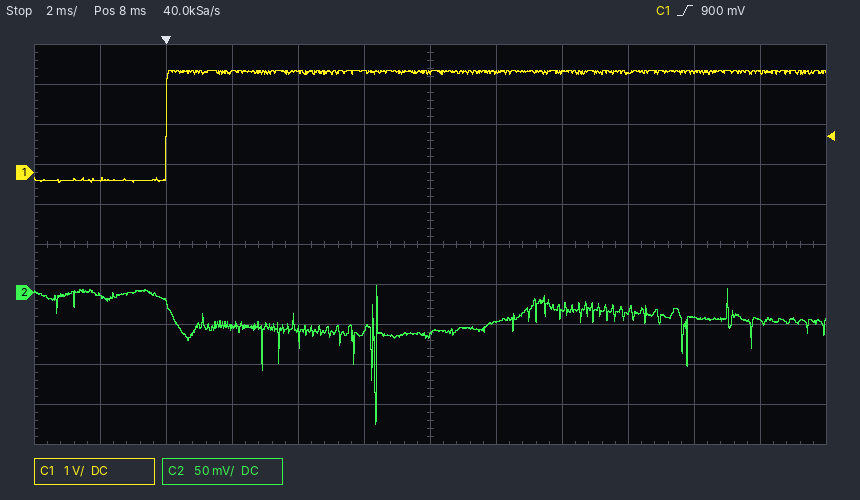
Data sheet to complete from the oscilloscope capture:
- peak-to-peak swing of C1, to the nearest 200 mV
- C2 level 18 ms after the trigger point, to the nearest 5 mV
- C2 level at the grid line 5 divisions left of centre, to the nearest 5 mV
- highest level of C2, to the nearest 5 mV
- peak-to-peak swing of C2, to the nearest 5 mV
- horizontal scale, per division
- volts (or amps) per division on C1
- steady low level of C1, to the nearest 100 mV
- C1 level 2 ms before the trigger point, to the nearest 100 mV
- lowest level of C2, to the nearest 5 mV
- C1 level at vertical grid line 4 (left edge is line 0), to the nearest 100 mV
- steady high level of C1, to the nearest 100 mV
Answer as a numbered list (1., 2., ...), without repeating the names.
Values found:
1. 2.8 V
2. -35 mV
3. -5 mV
4. 10 mV
5. 175 mV
6. 2 ms
7. 1 V
8. -200 mV
9. -200 mV
10. -165 mV
11. 2.5 V
12. 2.5 V
